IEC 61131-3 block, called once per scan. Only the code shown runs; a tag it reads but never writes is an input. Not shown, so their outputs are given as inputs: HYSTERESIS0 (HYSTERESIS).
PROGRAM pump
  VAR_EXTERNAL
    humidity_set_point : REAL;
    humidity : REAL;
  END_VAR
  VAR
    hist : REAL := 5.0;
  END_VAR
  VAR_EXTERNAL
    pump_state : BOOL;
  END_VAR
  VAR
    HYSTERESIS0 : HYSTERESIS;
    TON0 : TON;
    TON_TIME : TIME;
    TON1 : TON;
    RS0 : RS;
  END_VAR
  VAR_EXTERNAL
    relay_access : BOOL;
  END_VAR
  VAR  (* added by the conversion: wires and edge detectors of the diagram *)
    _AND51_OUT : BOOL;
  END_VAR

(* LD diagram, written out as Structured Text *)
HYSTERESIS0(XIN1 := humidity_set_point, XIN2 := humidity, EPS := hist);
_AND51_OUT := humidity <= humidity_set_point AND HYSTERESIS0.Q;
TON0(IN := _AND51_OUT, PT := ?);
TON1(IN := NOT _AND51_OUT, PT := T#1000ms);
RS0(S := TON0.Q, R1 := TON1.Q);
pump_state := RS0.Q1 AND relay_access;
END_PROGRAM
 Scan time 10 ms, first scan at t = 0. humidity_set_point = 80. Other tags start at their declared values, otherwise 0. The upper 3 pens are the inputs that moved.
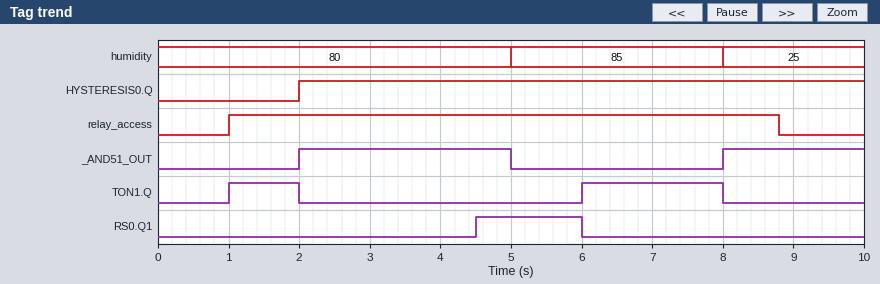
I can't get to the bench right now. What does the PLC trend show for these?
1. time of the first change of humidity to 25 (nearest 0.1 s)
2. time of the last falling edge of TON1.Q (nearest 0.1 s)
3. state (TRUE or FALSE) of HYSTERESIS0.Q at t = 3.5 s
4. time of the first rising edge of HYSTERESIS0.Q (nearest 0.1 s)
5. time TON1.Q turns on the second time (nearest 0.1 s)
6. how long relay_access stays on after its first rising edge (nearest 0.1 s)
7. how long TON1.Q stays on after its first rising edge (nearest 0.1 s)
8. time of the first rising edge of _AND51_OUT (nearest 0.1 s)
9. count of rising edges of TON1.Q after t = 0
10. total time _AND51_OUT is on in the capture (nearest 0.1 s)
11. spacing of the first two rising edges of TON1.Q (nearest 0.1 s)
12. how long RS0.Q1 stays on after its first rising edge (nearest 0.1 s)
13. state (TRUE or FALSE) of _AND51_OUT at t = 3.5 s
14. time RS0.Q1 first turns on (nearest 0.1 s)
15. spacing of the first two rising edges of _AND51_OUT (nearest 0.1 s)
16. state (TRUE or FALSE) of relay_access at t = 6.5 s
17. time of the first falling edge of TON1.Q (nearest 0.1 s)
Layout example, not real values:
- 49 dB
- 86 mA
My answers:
- 8.0 s
- 8.0 s
- TRUE
- 2.0 s
- 6.0 s
- 7.8 s
- 1.0 s
- 2.0 s
- 2
- 5.0 s
- 5.0 s
- 1.5 s
- TRUE
- 4.5 s
- 6.0 s
- TRUE
- 2.0 s
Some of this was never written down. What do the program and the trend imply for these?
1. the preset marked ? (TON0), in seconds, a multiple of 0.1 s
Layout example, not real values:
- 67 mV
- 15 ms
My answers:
- 2.5 s
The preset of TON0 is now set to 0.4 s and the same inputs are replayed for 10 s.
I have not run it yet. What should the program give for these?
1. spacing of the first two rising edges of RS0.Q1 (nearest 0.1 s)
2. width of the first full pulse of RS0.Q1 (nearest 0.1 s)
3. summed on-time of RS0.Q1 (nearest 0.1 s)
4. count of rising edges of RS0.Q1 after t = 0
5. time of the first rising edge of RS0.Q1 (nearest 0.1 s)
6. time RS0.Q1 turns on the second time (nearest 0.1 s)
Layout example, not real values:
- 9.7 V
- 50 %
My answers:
- 6.0 s
- 3.6 s
- 5.2 s
- 2
- 2.4 s
- 8.4 s
